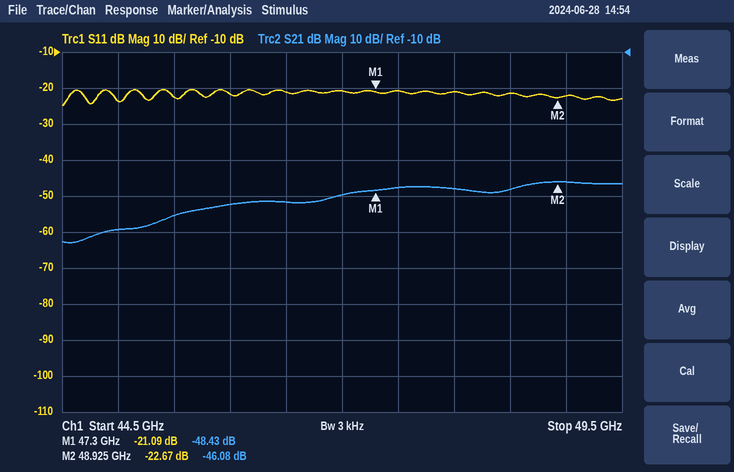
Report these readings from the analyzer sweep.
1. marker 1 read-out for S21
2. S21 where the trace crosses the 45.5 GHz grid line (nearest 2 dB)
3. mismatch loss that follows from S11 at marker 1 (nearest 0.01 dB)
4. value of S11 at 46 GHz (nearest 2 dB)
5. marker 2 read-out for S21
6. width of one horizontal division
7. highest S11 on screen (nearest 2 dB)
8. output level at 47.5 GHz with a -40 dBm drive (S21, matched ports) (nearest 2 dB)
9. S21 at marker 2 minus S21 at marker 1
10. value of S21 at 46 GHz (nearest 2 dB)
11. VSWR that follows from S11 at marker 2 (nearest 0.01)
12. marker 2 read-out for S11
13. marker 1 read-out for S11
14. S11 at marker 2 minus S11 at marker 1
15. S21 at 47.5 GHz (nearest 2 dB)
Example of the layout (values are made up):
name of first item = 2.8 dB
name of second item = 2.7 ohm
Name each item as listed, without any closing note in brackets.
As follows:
marker 1 read-out for S21 = -48.43 dB
S21 where the trace crosses the 45.5 GHz grid line = -56 dB
mismatch loss that follows from S11 at marker 1 = 0.03 dB
value of S11 at 46 GHz = -22 dB
marker 2 read-out for S21 = -46.08 dB
width of one horizontal division = 500 MHz
highest S11 on screen = -20 dB
output level at 47.5 GHz with a -40 dBm drive (S21, matched ports) = -88 dBm
S21 at marker 2 minus S21 at marker 1 = 2.35 dB
value of S21 at 46 GHz = -52 dB
VSWR that follows from S11 at marker 2 = 1.16
marker 2 read-out for S11 = -22.67 dB
marker 1 read-out for S11 = -21.09 dB
S11 at marker 2 minus S11 at marker 1 = -1.58 dB
S21 at 47.5 GHz = -48 dB
